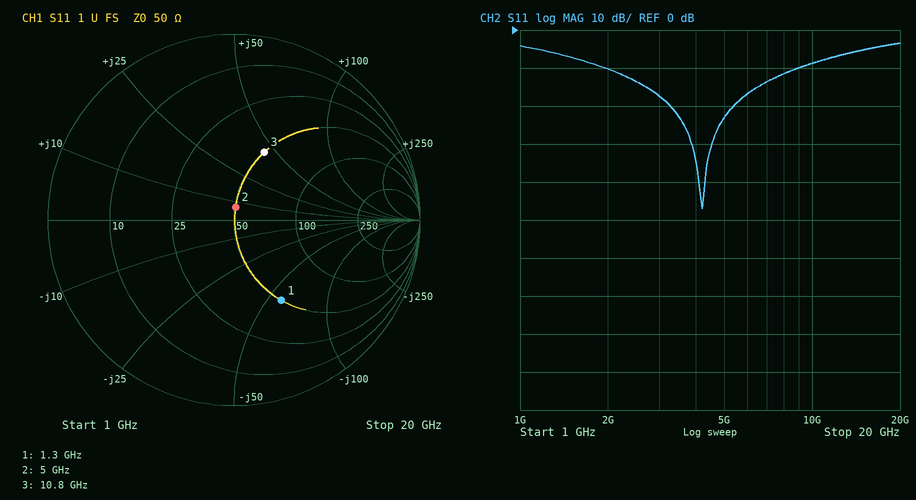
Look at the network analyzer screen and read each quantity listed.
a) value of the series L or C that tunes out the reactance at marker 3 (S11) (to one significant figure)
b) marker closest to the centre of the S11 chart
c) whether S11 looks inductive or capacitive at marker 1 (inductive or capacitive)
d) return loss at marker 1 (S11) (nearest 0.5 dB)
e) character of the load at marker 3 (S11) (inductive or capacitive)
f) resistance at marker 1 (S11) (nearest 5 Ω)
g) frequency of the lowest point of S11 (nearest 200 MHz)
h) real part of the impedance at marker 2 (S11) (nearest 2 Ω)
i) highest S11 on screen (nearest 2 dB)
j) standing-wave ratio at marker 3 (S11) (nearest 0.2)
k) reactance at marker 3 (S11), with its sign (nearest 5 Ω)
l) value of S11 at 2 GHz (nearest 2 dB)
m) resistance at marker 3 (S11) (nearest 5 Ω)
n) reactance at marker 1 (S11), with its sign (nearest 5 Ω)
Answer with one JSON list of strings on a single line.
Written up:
["300 fF", "marker 2", "capacitive", "6.0 dB", "inductive", "50 Ω", "4.2 GHz", "50 Ω", "-4 dB", "2.4", "+45 Ω", "-10 dB", "50 Ω", "-60 Ω"]
